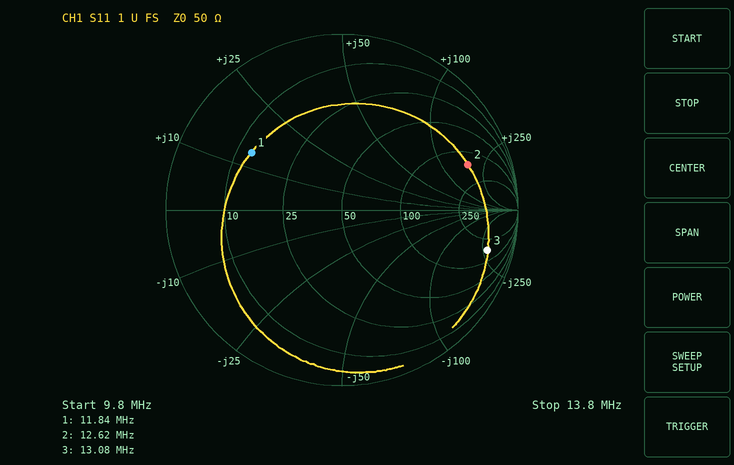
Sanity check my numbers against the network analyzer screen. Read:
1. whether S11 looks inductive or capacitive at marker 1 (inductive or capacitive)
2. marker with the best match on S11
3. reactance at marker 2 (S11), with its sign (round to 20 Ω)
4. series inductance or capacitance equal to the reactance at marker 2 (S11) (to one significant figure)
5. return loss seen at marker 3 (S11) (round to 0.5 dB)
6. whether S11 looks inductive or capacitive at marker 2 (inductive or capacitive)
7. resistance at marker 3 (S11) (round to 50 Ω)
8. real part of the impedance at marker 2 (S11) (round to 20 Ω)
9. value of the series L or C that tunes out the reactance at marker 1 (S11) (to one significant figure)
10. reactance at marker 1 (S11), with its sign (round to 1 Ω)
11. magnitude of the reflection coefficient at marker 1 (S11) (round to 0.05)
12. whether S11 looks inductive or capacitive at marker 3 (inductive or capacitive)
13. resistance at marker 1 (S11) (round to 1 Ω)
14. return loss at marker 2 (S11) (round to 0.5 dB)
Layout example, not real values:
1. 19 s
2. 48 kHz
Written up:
1. inductive
2. marker 1
3. +180 Ω
4. 2 µH
5. 1.5 dB
6. inductive
7. 150 Ω
8. 140 Ω
9. 1.0 nF
10. +14 Ω
11. 0.60
12. capacitive
13. 13 Ω
14. 2.5 dB
